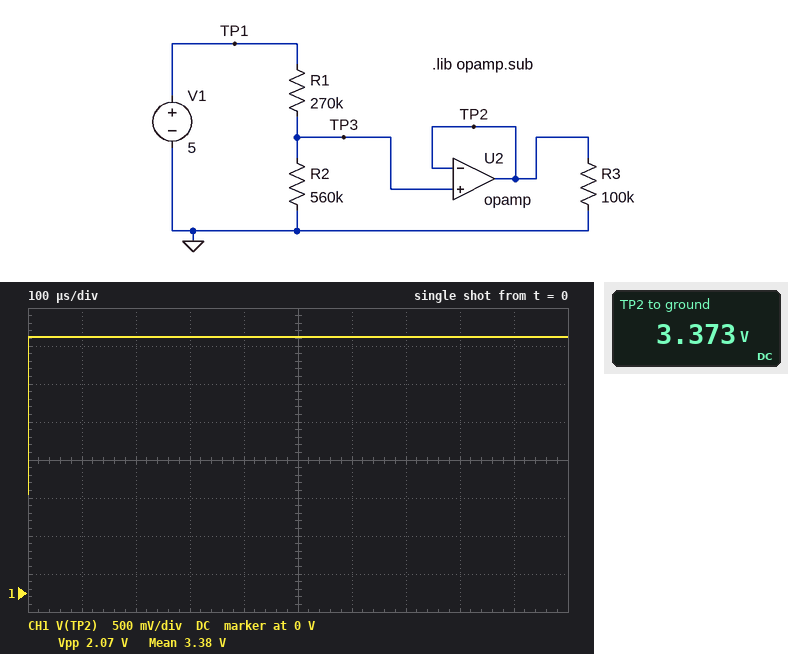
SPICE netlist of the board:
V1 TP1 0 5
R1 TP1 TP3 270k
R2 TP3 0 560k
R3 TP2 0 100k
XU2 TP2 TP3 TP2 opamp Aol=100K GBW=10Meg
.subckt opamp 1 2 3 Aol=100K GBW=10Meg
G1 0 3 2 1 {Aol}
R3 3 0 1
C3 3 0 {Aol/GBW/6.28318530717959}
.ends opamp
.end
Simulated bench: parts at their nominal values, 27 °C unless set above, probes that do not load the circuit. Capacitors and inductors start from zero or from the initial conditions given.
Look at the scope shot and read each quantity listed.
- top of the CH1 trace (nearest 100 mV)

3.4 V
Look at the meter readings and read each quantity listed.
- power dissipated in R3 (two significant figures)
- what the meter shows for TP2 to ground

110 µW
3.373 V
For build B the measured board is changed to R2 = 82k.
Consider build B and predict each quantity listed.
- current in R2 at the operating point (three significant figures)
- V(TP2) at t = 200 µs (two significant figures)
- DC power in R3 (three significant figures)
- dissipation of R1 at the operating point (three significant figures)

14.2 µA
1.2 V
13.6 µW
54.5 µW
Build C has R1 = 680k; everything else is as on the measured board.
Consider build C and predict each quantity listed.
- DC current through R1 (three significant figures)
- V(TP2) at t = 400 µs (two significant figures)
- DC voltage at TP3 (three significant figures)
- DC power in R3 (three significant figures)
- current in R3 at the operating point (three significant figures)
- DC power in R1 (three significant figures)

4.03 µA
2.3 V
2.26 V
51.0 µW
22.6 µA
11.1 µW
